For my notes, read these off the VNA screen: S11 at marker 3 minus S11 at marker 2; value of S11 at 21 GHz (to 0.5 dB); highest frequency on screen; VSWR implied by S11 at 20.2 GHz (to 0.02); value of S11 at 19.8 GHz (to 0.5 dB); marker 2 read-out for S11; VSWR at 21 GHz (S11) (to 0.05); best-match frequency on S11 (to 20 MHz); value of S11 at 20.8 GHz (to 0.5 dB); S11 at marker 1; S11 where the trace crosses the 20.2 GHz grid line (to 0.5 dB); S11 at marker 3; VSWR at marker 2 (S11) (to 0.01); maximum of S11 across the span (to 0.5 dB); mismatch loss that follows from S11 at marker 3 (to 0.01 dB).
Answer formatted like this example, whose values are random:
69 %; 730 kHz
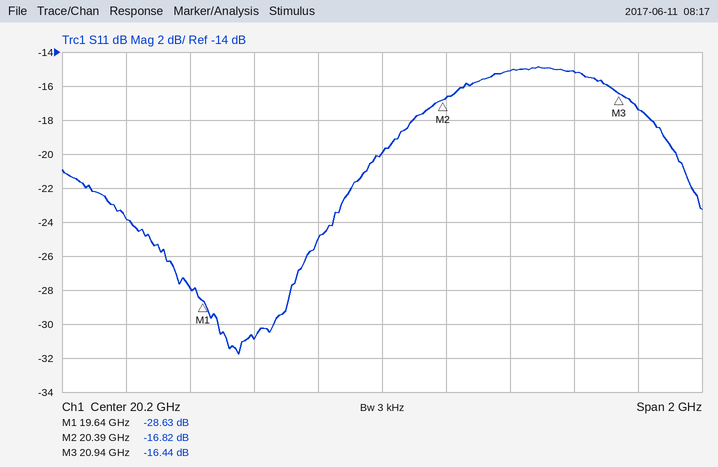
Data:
0.38 dB; -17.5 dB; 21.2 GHz; 1.22; -31.0 dB; -16.82 dB; 1.30; 19.76 GHz; -15.0 dB; -28.63 dB; -20.0 dB; -16.44 dB; 1.34; -15.0 dB; 0.10 dB
